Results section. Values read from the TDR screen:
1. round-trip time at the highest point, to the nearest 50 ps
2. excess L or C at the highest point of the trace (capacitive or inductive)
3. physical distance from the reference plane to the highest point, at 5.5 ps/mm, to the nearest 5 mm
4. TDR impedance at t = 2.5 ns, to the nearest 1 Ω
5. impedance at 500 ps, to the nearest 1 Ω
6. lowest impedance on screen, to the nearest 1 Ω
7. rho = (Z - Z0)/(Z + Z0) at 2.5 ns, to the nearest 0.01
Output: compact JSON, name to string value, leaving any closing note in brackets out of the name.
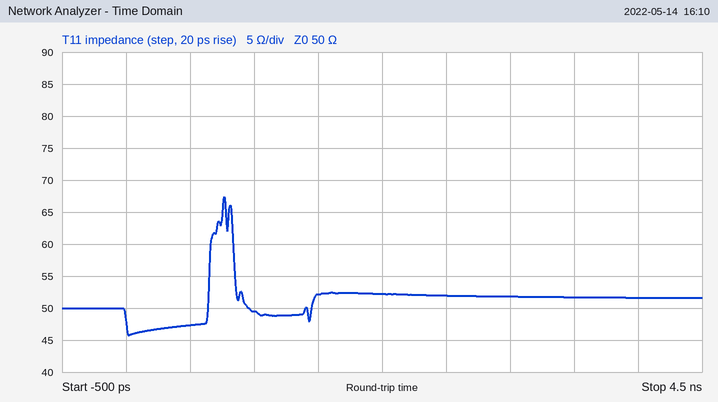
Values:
{"round-trip time at the highest point, to the nearest 50 ps": "750 ps", "excess L or C at the highest point of the trace": "inductive", "physical distance from the reference plane to the highest point, at 5.5 ps/mm, to the nearest 5 mm": "70 mm", "TDR impedance at t = 2.5 ns, to the nearest 1 Ω": "52 Ω", "impedance at 500 ps, to the nearest 1 Ω": "47 Ω", "lowest impedance on screen, to the nearest 1 Ω": "46 Ω", "rho = (Z - Z0)/(Z + Z0) at 2.5 ns, to the nearest 0.01": "+0.02"}
